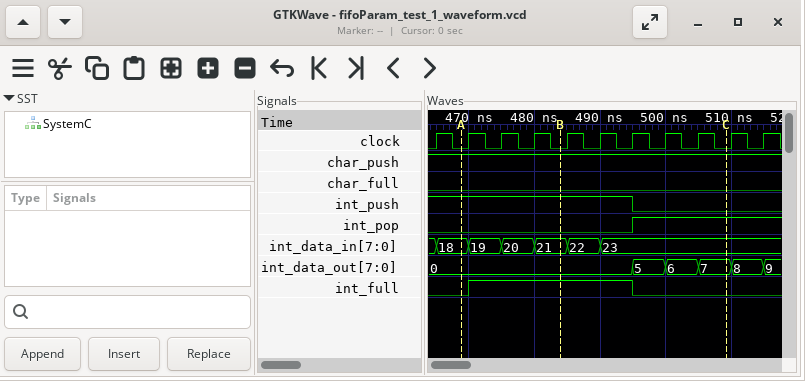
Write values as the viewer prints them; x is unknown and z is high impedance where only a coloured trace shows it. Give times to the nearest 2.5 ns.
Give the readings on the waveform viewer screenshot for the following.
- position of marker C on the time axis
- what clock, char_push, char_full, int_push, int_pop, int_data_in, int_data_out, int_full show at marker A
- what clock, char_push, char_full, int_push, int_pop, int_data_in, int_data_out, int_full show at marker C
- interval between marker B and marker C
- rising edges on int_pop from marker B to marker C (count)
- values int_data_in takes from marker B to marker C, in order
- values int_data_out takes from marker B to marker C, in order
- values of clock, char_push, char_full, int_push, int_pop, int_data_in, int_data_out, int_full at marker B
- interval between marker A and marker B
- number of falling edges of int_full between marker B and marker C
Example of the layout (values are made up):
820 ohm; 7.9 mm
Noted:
510 ns; clock=0, char_push=1, char_full=0, int_push=1, int_pop=0, int_data_in=18, int_data_out=0, int_full=0; clock=0, char_push=1, char_full=0, int_push=0, int_pop=1, int_data_in=23, int_data_out=7, int_full=0; 25 ns; 1; 21, 22, 23; 0, 5, 6, 7; clock=0, char_push=1, char_full=0, int_push=1, int_pop=0, int_data_in=21, int_data_out=0, int_full=1; 15 ns; 1
